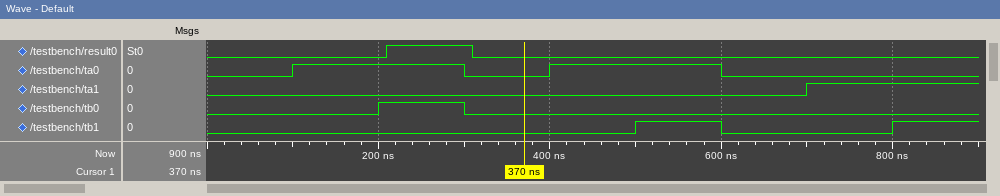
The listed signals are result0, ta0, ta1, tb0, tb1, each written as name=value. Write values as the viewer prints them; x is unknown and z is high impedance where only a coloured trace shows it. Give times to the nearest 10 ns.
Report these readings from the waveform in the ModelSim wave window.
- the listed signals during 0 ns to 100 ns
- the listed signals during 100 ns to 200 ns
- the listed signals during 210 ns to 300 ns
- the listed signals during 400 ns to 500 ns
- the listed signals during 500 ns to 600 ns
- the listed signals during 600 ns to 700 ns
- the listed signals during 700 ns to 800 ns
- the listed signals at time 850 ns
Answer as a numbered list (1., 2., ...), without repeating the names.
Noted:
1. result0=0, ta0=0, ta1=0, tb0=0, tb1=0
2. result0=0, ta0=1, ta1=0, tb0=0, tb1=0
3. result0=1, ta0=1, ta1=0, tb0=1, tb1=0
4. result0=0, ta0=1, ta1=0, tb0=0, tb1=0
5. result0=0, ta0=1, ta1=0, tb0=0, tb1=1
6. result0=0, ta0=0, ta1=0, tb0=0, tb1=0
7. result0=0, ta0=0, ta1=1, tb0=0, tb1=0
8. result0=0, ta0=0, ta1=1, tb0=0, tb1=1
